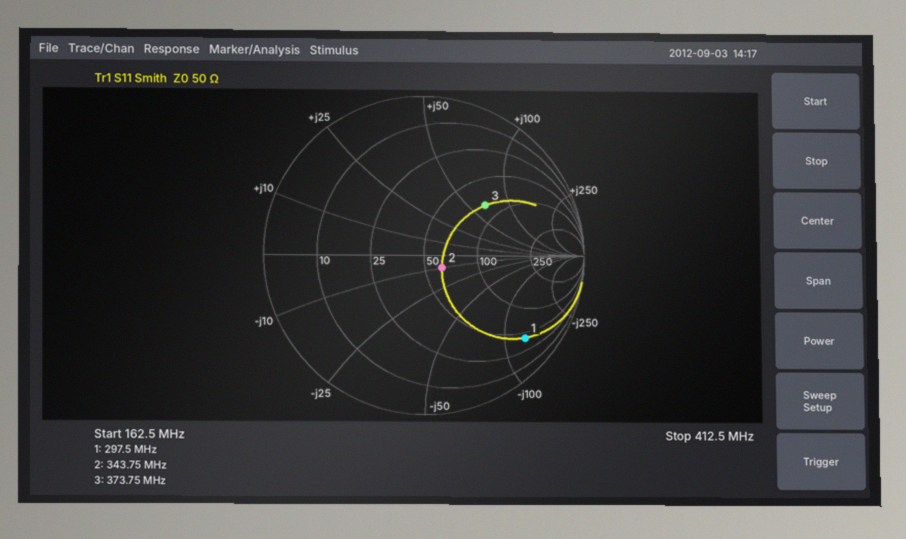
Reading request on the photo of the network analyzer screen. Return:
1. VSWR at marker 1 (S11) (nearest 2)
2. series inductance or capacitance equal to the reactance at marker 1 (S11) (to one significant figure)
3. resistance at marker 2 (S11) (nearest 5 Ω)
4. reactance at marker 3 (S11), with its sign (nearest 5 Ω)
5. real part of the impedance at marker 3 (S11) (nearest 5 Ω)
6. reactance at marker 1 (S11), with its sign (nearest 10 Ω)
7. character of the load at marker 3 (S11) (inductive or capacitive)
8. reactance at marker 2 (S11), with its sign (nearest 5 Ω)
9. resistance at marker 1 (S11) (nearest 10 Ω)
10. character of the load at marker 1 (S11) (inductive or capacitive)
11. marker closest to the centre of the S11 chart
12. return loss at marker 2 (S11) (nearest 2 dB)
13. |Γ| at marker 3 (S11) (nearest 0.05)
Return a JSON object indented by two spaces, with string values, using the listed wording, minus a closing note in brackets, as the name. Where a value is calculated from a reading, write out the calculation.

{
  "VSWR at marker 1 (S11)": "10",
  "series inductance or capacitance equal to the reactance at marker 1 (S11)": "C = 1/(2π × 297.5 MHz × 130 Ω) ≈ 4 pF",
  "resistance at marker 2 (S11)": "60 Ω",
  "reactance at marker 3 (S11), with its sign": "+65 Ω",
  "real part of the impedance at marker 3 (S11)": "80 Ω",
  "reactance at marker 1 (S11), with its sign": "-130 Ω",
  "character of the load at marker 3 (S11)": "inductive",
  "reactance at marker 2 (S11), with its sign": "-10 Ω",
  "resistance at marker 1 (S11)": "40 Ω",
  "character of the load at marker 1 (S11)": "capacitive",
  "marker closest to the centre of the S11 chart": "marker 2",
  "return loss at marker 2 (S11)": "18 dB",
  "|Γ| at marker 3 (S11)": "0.50"
}
